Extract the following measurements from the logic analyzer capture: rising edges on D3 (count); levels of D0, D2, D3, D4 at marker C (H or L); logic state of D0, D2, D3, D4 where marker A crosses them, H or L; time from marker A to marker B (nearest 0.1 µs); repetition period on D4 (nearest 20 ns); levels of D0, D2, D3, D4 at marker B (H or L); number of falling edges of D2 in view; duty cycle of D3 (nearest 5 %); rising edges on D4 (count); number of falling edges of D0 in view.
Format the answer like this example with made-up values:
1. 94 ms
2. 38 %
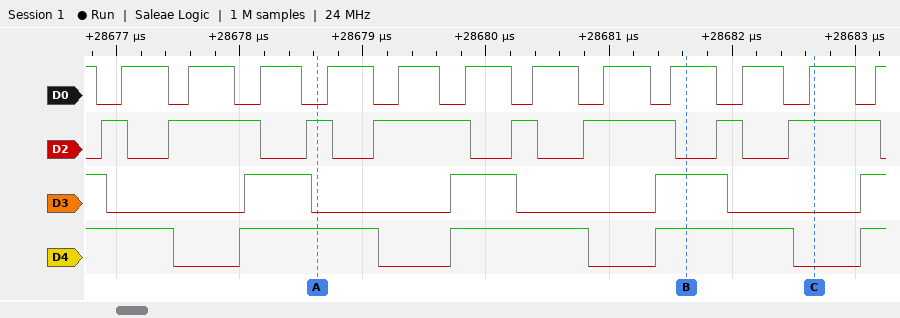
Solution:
1. 4
2. D0=H, D2=H, D3=L, D4=L
3. D0=L, D2=H, D3=L, D4=H
4. 3 µs
5. 1680 ns
6. D0=H, D2=L, D3=H, D4=H
7. 8
8. 35 %
9. 4
10. 12
